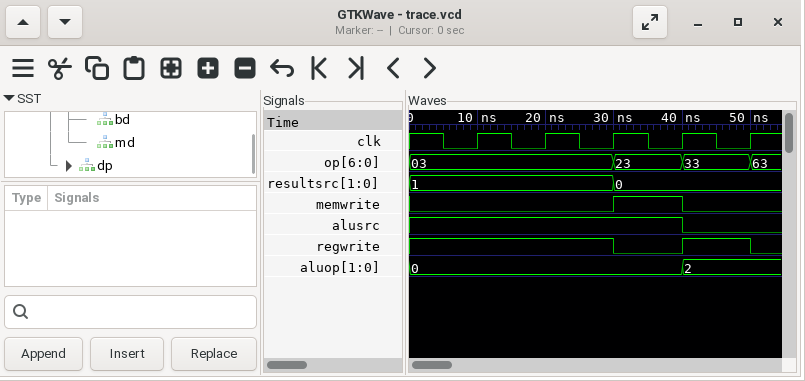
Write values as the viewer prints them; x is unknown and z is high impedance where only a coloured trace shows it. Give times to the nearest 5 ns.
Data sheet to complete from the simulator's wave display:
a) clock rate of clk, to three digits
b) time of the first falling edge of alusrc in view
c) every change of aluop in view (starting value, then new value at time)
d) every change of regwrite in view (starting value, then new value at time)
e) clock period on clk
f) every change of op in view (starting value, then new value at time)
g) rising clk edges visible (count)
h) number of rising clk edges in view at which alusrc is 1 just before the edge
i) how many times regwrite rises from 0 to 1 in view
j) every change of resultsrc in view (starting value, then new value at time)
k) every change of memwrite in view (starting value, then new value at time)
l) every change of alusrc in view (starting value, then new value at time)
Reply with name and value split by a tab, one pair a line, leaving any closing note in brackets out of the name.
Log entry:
clock rate of clk, to three digits	100 MHz
time of the first falling edge of alusrc in view	40 ns
every change of aluop in view	0, 2 at 40 ns
every change of regwrite in view	1, 0 at 30 ns, 1 at 40 ns, 0 at 50 ns
clock period on clk	10 ns
every change of op in view	03, 23 at 30 ns, 33 at 40 ns, 63 at 50 ns
rising clk edges visible	5
number of rising clk edges in view at which alusrc is 1 just before the edge	4
how many times regwrite rises from 0 to 1 in view	1
every change of resultsrc in view	1, 0 at 30 ns
every change of memwrite in view	0, 1 at 30 ns, 0 at 40 ns
every change of alusrc in view	1, 0 at 40 ns
